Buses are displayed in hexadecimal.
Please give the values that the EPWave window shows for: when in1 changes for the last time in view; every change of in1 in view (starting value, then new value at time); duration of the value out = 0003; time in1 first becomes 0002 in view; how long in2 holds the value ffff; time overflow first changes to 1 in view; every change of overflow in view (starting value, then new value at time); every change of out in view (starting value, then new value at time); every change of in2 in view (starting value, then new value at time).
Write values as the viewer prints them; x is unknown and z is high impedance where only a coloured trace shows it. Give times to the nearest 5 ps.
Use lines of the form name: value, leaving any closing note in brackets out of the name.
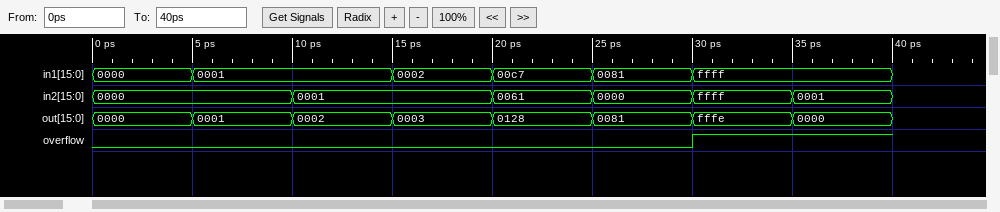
when in1 changes for the last time in view: 30 ps
every change of in1 in view: 0000, 0001 at 5 ps, 0002 at 15 ps, 00c7 at 20 ps, 0081 at 25 ps, ffff at 30 ps
duration of the value out = 0003: 5 ps
time in1 first becomes 0002 in view: 15 ps
how long in2 holds the value ffff: 5 ps
time overflow first changes to 1 in view: 30 ps
every change of overflow in view: 0, 1 at 30 ps
every change of out in view: 0000, 0001 at 5 ps, 0002 at 10 ps, 0003 at 15 ps, 0128 at 20 ps, 0081 at 25 ps, fffe at 30 ps, 0000 at 35 ps
every change of in2 in view: 0000, 0001 at 10 ps, 0061 at 20 ps, 0000 at 25 ps, ffff at 30 ps, 0001 at 35 ps
